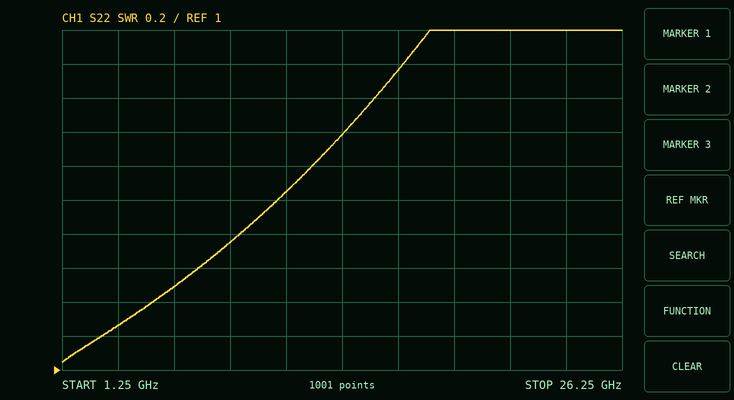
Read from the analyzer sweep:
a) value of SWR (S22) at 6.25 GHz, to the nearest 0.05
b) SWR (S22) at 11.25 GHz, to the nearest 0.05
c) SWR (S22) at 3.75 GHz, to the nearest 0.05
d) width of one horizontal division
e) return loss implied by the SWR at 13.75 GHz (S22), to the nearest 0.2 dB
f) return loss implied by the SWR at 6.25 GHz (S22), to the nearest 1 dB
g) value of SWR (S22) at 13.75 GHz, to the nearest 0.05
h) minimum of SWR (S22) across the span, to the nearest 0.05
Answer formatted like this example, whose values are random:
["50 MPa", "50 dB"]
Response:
["1.50", "2.05", "1.25", "2.5 GHz", "7.8 dB", "14 dB", "2.40", "1.05"]
